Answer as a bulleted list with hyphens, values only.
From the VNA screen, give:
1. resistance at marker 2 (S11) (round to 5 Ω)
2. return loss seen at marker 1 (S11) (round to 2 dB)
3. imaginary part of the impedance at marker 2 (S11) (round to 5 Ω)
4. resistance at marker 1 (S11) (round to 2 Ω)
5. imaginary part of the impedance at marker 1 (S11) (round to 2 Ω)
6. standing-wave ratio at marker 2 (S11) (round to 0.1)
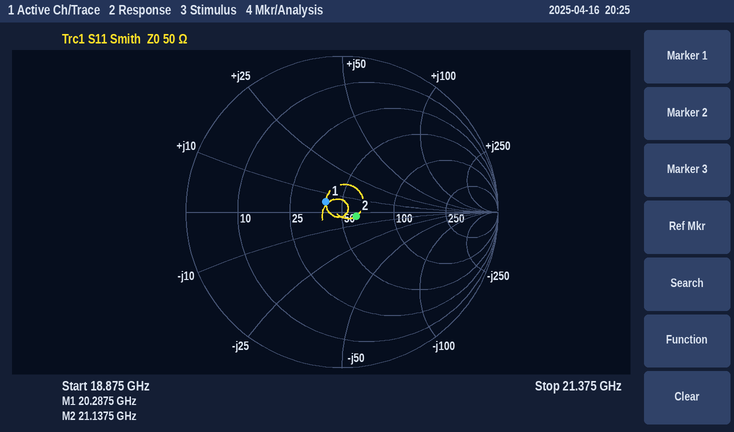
- 60 Ω
- 18 dB
- -5 Ω
- 40 Ω
- +6 Ω
- 1.2
